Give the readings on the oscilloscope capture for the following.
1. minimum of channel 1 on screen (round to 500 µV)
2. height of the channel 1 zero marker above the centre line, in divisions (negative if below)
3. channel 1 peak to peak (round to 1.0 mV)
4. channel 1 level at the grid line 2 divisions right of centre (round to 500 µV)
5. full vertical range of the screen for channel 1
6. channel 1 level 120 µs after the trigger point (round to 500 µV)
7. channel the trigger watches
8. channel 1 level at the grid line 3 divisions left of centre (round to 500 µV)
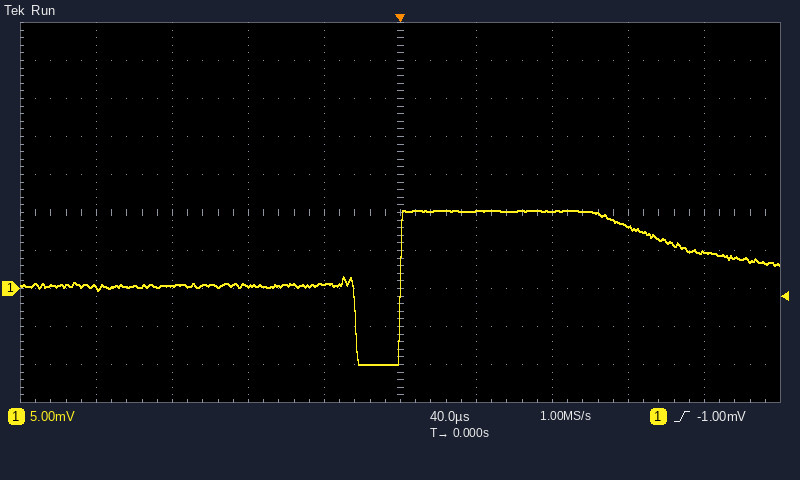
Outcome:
-10.0 mV
-2.0 div
20.0 mV
10.0 mV
50 mV
8.0 mV
channel 1
500 µV
